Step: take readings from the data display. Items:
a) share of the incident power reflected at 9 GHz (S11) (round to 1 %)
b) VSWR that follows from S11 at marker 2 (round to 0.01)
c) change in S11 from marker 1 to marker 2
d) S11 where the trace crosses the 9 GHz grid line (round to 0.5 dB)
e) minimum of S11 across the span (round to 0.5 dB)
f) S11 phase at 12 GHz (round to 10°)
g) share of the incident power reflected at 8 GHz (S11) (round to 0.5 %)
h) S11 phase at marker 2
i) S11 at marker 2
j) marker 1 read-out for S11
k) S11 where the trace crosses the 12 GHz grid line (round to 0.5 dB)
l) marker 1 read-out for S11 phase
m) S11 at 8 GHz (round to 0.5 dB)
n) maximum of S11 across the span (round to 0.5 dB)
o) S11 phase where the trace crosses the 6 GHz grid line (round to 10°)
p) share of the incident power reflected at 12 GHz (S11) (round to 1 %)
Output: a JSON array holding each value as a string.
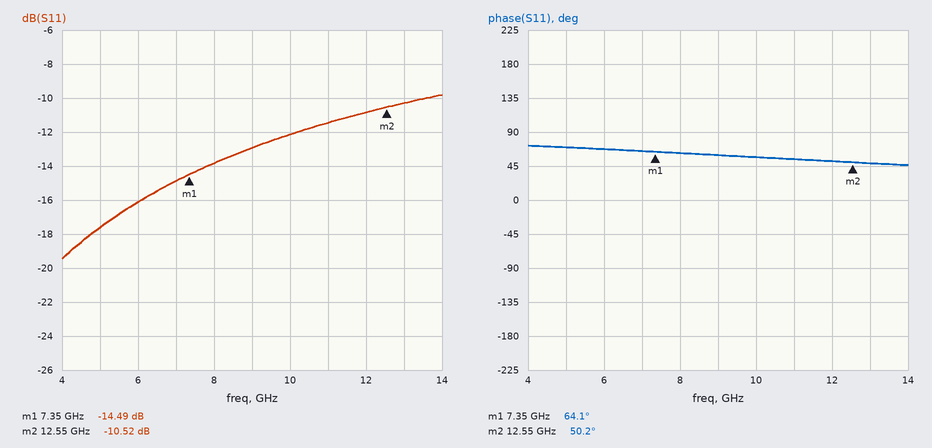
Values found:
["5 %", "1.85", "3.97 dB", "-13.0 dB", "-19.5 dB", "50°", "4.0 %", "50.2°", "-10.52 dB", "-14.49 dB", "-11.0 dB", "64.1°", "-14.0 dB", "-10.0 dB", "70°", "8 %"]
